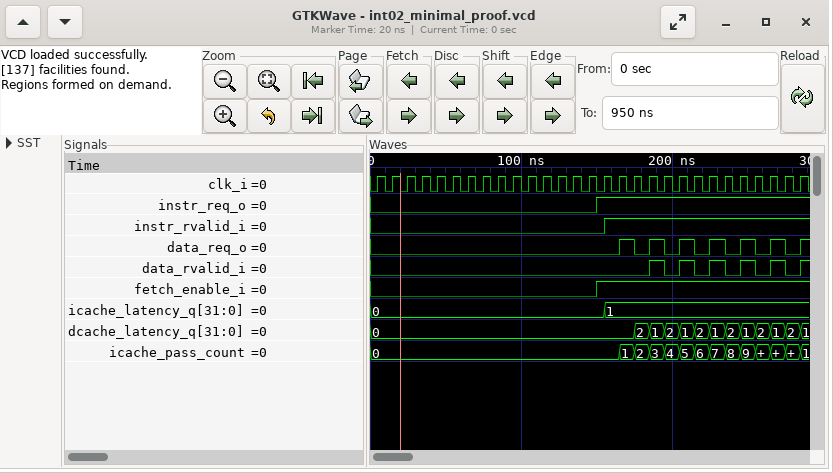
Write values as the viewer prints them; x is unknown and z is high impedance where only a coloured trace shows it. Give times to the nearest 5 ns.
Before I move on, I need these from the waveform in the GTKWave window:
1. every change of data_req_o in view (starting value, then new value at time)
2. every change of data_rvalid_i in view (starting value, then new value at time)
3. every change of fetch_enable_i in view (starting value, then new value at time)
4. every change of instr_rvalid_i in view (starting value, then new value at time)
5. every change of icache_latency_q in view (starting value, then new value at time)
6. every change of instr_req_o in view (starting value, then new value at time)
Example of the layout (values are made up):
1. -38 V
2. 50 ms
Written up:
1. 0, 1 at 165 ns, 0 at 175 ns, 1 at 185 ns, 0 at 195 ns, 1 at 205 ns, 0 at 215 ns, 1 at 225 ns, 0 at 235 ns, 1 at 245 ns, 0 at 255 ns, 1 at 265 ns, 0 at 275 ns, 1 at 285 ns
2. 0, 1 at 185 ns, 0 at 195 ns, 1 at 205 ns, 0 at 215 ns, 1 at 225 ns, 0 at 235 ns, 1 at 245 ns, 0 at 255 ns, 1 at 265 ns, 0 at 275 ns, 1 at 285 ns
3. 0, 1 at 150 ns
4. 0, 1 at 155 ns
5. 0, 1 at 155 ns
6. 0, 1 at 150 ns
